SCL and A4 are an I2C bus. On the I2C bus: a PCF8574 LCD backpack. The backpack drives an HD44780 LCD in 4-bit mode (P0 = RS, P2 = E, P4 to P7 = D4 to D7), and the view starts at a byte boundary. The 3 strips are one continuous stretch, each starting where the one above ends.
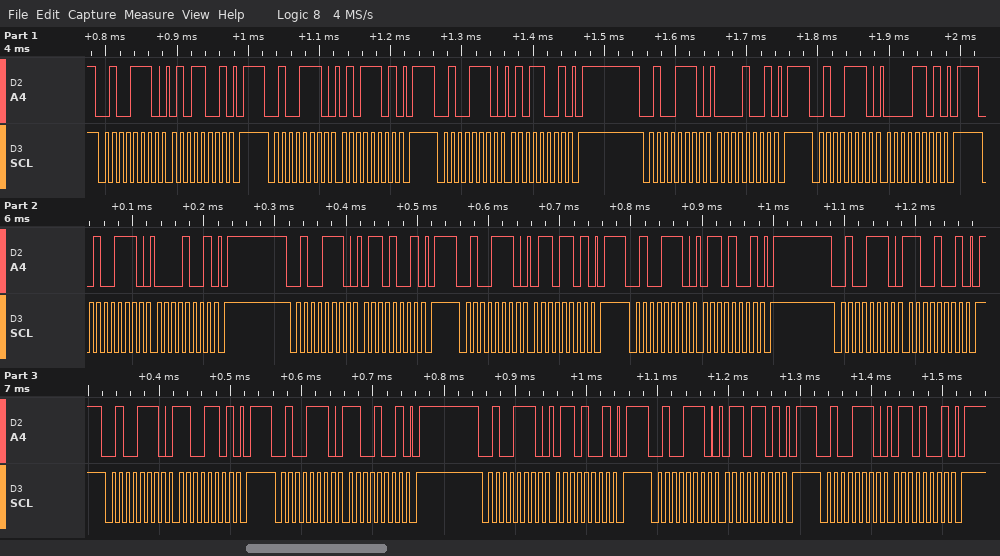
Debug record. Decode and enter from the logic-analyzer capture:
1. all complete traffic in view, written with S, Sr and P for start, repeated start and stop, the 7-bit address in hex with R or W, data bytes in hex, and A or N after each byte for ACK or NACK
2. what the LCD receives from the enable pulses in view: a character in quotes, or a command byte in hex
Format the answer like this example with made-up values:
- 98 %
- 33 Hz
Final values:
- S 27W A 59 A P S 27W A 5D A P S 27W A 59 A P S 27W A 09 A P S 27W A 0D A P S 27W A 09 A P S 27W A 69 A P S 27W A 6D A P S 27W A 69 A P S 27W A C9 A P S 27W A CD A P S 27W A C9 A P S 27W A 69 A P S 27W A 6D A P S 27W A 69 A P
- 'P' 'l'
